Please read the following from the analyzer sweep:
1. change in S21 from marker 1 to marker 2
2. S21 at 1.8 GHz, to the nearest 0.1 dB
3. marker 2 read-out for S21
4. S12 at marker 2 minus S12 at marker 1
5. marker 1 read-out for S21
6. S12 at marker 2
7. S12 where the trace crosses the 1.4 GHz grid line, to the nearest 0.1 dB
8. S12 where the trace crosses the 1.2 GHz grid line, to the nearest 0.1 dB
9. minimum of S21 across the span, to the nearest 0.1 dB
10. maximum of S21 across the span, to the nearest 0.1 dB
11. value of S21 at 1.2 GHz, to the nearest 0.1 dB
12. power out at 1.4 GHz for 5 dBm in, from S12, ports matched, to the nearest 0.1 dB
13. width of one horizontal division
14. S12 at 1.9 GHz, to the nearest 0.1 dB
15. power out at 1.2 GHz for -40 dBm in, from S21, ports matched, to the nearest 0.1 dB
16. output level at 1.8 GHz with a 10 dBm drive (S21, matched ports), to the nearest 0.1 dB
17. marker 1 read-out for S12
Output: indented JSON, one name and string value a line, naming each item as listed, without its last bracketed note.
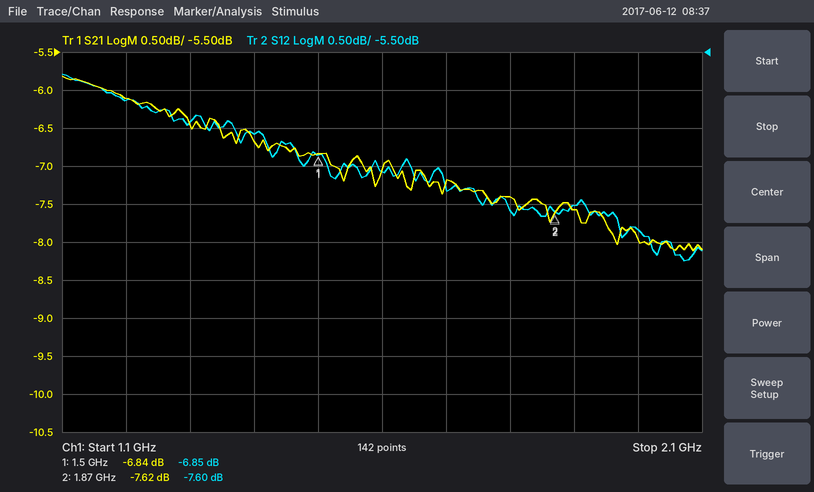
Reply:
{
  "change in S21 from marker 1 to marker 2": "-0.78 dB",
  "S21 at 1.8 GHz, to the nearest 0.1 dB": "-7.4 dB",
  "marker 2 read-out for S21": "-7.62 dB",
  "S12 at marker 2 minus S12 at marker 1": "-0.75 dB",
  "marker 1 read-out for S21": "-6.84 dB",
  "S12 at marker 2": "-7.60 dB",
  "S12 where the trace crosses the 1.4 GHz grid line, to the nearest 0.1 dB": "-6.6 dB",
  "S12 where the trace crosses the 1.2 GHz grid line, to the nearest 0.1 dB": "-6.1 dB",
  "minimum of S21 across the span, to the nearest 0.1 dB": "-8.1 dB",
  "maximum of S21 across the span, to the nearest 0.1 dB": "-5.8 dB",
  "value of S21 at 1.2 GHz, to the nearest 0.1 dB": "-6.1 dB",
  "power out at 1.4 GHz for 5 dBm in, from S12, ports matched, to the nearest 0.1 dB": "-1.6 dBm",
  "width of one horizontal division": "100 MHz",
  "S12 at 1.9 GHz, to the nearest 0.1 dB": "-7.5 dB",
  "power out at 1.2 GHz for -40 dBm in, from S21, ports matched, to the nearest 0.1 dB": "-46.1 dBm",
  "output level at 1.8 GHz with a 10 dBm drive (S21, matched ports), to the nearest 0.1 dB": "2.6 dBm",
  "marker 1 read-out for S12": "-6.85 dB"
}
